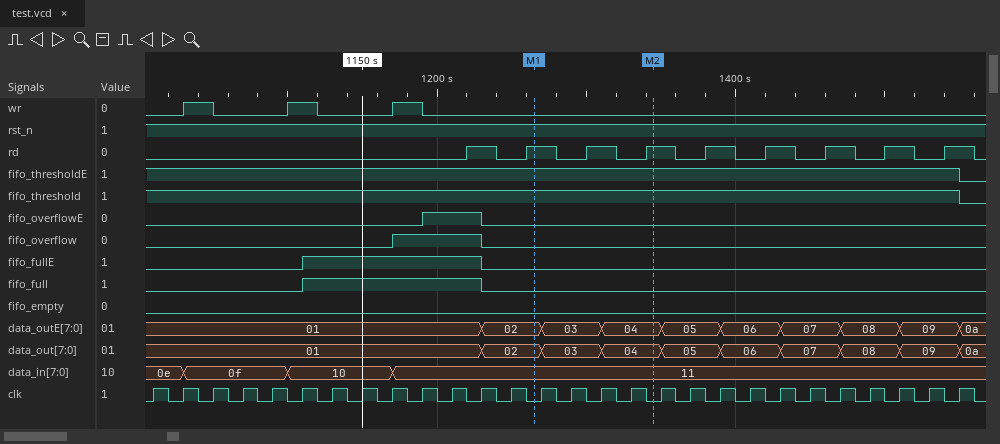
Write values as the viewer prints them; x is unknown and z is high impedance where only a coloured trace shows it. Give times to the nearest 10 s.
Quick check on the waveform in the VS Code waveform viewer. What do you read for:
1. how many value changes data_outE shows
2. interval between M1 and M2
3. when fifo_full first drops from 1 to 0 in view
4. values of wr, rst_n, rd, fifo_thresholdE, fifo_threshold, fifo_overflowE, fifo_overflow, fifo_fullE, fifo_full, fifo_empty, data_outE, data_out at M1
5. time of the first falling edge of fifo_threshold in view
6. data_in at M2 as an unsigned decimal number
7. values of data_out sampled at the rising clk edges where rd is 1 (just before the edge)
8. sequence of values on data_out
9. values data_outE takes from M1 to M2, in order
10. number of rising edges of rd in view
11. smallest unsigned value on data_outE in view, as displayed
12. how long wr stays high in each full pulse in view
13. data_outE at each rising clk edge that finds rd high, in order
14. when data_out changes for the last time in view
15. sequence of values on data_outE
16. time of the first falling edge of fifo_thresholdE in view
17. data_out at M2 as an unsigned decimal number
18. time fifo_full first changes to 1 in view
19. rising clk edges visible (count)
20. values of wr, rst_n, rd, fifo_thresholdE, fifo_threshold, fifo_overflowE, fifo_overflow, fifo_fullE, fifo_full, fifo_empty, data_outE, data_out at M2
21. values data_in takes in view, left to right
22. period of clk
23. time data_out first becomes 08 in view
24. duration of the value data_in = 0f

9
80 s
1230 s
wr=0, rst_n=1, rd=1, fifo_thresholdE=1, fifo_threshold=1, fifo_overflowE=0, fifo_overflow=0, fifo_fullE=0, fifo_full=0, fifo_empty=0, data_outE=02, data_out=02
1550 s
17
01, 02, 03, 04, 05, 06, 07, 08, 09
01, 02, 03, 04, 05, 06, 07, 08, 09, 0a
02, 03, 04
9
01
20 s, 20 s, 20 s
01, 02, 03, 04, 05, 06, 07, 08, 09
1550 s
01, 02, 03, 04, 05, 06, 07, 08, 09, 0a
1550 s
4
1110 s
28
wr=0, rst_n=1, rd=1, fifo_thresholdE=1, fifo_threshold=1, fifo_overflowE=0, fifo_overflow=0, fifo_fullE=0, fifo_full=0, fifo_empty=0, data_outE=04, data_out=04
0e, 0f, 10, 11
20 s
1470 s
70 s
